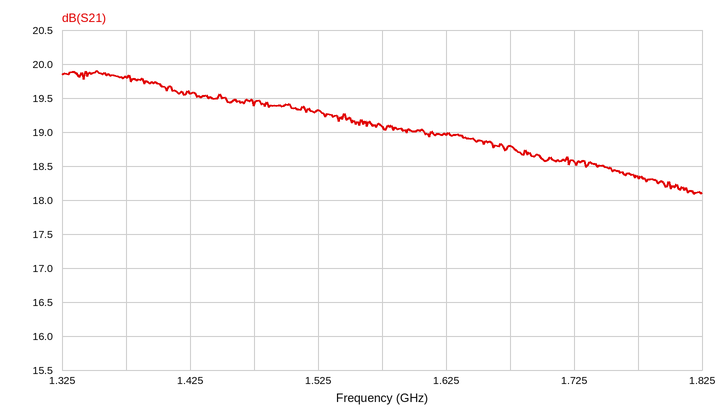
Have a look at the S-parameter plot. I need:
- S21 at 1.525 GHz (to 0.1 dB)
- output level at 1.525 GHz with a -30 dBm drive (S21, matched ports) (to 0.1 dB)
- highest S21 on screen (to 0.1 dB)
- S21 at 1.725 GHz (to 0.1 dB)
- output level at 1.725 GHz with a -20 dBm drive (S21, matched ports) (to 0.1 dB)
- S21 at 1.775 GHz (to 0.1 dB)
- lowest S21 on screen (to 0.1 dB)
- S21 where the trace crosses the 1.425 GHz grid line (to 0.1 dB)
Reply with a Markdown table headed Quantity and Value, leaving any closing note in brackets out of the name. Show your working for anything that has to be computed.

| Quantity | Value |
|---|---|
| S21 at 1.525 GHz | 19.3 dB |
| output level at 1.525 GHz with a -30 dBm drive (S21, matched ports) | -30 dBm + (19.3 dB) = -10.7 dBm |
| highest S21 on screen | 19.9 dB |
| S21 at 1.725 GHz | 18.6 dB |
| output level at 1.725 GHz with a -20 dBm drive (S21, matched ports) | -20 dBm + (18.6 dB) = -1.4 dBm |
| S21 at 1.775 GHz | 18.3 dB |
| lowest S21 on screen | 18.1 dB |
| S21 where the trace crosses the 1.425 GHz grid line | 19.6 dB |
